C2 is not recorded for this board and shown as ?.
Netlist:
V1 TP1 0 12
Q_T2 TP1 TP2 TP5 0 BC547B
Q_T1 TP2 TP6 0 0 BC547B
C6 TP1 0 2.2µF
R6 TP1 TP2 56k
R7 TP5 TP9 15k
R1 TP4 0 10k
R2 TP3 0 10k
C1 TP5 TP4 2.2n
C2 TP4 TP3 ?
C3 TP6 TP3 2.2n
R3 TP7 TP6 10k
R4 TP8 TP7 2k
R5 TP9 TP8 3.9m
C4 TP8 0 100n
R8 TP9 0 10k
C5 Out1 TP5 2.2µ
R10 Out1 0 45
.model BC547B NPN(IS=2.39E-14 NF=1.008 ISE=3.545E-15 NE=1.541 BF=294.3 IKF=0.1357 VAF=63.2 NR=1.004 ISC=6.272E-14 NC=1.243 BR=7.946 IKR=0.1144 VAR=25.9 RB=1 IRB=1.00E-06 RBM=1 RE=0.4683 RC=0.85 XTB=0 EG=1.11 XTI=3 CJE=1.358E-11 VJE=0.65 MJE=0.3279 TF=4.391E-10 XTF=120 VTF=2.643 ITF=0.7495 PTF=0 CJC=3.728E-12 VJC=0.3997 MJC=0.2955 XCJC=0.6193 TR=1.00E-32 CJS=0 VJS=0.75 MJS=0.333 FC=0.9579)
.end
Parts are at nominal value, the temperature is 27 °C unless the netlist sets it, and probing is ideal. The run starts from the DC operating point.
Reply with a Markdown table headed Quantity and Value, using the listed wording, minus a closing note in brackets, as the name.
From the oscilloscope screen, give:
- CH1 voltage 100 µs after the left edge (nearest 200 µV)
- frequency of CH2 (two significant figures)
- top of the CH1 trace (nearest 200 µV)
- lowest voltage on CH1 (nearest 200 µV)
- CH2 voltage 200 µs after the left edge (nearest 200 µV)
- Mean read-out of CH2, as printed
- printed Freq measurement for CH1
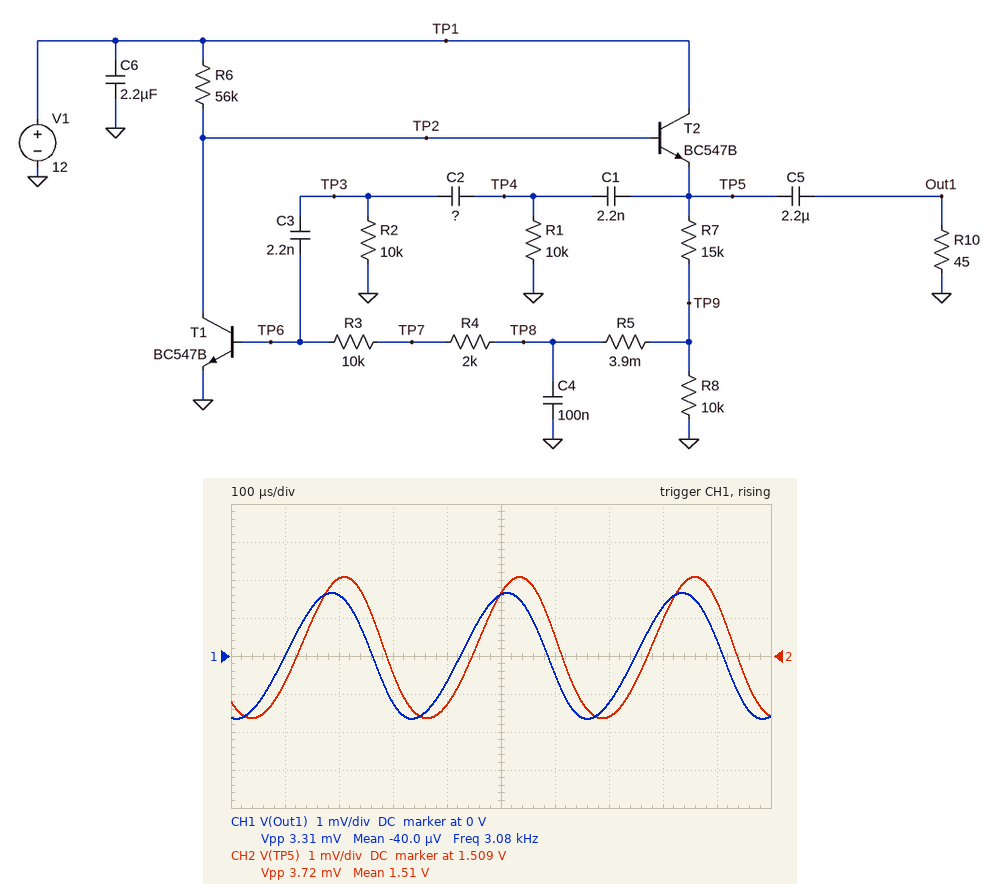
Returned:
| Quantity | Value |
|---|---|
| CH1 voltage 100 µs after the left edge | 0 V |
| frequency of CH2 | 3.1 kHz |
| top of the CH1 trace | 1.6 mV |
| lowest voltage on CH1 | -1.6 mV |
| CH2 voltage 200 µs after the left edge | 1.5110 V |
| Mean read-out of CH2, as printed | 1.51 V |
| printed Freq measurement for CH1 | 3.08 kHz |
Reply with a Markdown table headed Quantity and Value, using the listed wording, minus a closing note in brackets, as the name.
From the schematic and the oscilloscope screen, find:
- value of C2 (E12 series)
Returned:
| Quantity | Value |
|---|---|
| value of C2 | 1.8 nF |
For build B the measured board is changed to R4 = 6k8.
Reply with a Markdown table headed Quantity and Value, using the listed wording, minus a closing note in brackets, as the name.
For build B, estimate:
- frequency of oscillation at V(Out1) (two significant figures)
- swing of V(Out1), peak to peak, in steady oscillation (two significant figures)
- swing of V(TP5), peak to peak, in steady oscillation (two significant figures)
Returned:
| Quantity | Value |
|---|---|
| frequency of oscillation at V(Out1) | 2.7 kHz |
| swing of V(Out1), peak to peak, in steady oscillation | 3.9 mV |
| swing of V(TP5), peak to peak, in steady oscillation | 4.5 mV |
